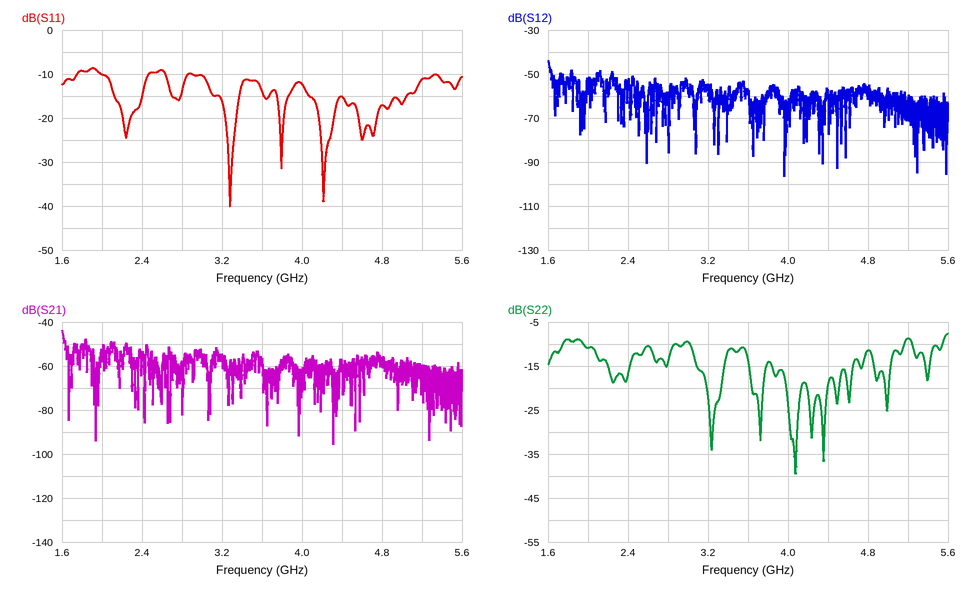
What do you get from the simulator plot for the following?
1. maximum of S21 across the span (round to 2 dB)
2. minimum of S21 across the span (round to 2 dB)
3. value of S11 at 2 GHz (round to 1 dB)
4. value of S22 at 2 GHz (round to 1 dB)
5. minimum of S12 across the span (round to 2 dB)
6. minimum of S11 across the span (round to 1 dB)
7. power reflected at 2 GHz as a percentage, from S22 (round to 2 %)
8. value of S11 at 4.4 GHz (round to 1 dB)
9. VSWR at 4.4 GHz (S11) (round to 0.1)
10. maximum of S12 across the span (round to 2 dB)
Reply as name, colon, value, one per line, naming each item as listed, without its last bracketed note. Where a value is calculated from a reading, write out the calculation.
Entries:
maximum of S21 across the span: -44 dB
minimum of S21 across the span: -96 dB
value of S11 at 2 GHz: -10 dB
value of S22 at 2 GHz: -11 dB
minimum of S12 across the span: -96 dB
minimum of S11 across the span: -40 dB
power reflected at 2 GHz as a percentage, from S22: 10^(-11/10) ≈ 8 %
value of S11 at 4.4 GHz: -15 dB
VSWR at 4.4 GHz (S11): |Γ| = 10^(-15/20) = 0.1778; VSWR = (1 + 0.1778)/(1 − 0.1778) ≈ 1.4
maximum of S12 across the span: -44 dB
